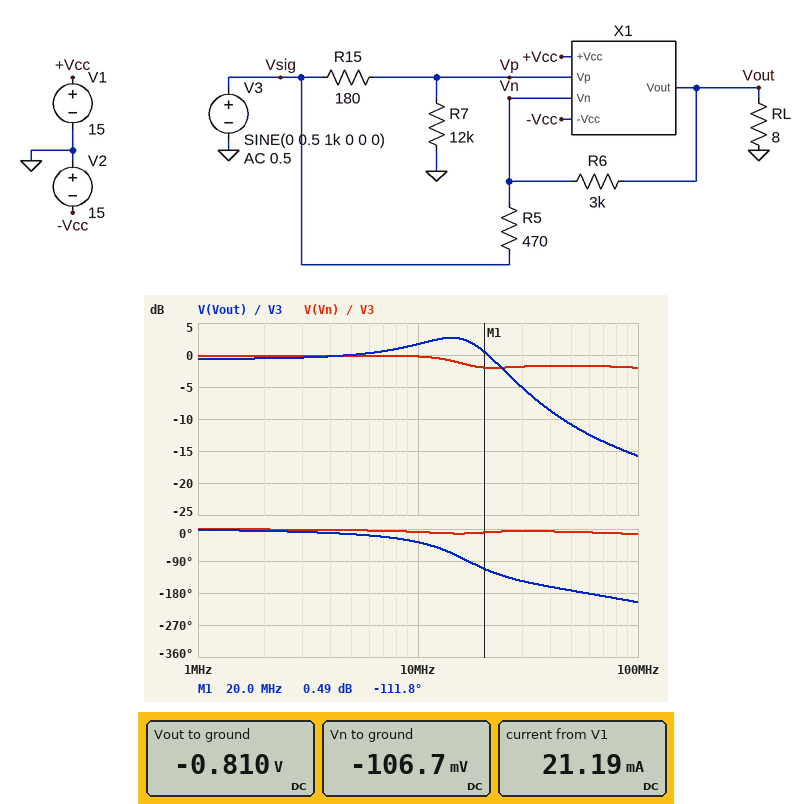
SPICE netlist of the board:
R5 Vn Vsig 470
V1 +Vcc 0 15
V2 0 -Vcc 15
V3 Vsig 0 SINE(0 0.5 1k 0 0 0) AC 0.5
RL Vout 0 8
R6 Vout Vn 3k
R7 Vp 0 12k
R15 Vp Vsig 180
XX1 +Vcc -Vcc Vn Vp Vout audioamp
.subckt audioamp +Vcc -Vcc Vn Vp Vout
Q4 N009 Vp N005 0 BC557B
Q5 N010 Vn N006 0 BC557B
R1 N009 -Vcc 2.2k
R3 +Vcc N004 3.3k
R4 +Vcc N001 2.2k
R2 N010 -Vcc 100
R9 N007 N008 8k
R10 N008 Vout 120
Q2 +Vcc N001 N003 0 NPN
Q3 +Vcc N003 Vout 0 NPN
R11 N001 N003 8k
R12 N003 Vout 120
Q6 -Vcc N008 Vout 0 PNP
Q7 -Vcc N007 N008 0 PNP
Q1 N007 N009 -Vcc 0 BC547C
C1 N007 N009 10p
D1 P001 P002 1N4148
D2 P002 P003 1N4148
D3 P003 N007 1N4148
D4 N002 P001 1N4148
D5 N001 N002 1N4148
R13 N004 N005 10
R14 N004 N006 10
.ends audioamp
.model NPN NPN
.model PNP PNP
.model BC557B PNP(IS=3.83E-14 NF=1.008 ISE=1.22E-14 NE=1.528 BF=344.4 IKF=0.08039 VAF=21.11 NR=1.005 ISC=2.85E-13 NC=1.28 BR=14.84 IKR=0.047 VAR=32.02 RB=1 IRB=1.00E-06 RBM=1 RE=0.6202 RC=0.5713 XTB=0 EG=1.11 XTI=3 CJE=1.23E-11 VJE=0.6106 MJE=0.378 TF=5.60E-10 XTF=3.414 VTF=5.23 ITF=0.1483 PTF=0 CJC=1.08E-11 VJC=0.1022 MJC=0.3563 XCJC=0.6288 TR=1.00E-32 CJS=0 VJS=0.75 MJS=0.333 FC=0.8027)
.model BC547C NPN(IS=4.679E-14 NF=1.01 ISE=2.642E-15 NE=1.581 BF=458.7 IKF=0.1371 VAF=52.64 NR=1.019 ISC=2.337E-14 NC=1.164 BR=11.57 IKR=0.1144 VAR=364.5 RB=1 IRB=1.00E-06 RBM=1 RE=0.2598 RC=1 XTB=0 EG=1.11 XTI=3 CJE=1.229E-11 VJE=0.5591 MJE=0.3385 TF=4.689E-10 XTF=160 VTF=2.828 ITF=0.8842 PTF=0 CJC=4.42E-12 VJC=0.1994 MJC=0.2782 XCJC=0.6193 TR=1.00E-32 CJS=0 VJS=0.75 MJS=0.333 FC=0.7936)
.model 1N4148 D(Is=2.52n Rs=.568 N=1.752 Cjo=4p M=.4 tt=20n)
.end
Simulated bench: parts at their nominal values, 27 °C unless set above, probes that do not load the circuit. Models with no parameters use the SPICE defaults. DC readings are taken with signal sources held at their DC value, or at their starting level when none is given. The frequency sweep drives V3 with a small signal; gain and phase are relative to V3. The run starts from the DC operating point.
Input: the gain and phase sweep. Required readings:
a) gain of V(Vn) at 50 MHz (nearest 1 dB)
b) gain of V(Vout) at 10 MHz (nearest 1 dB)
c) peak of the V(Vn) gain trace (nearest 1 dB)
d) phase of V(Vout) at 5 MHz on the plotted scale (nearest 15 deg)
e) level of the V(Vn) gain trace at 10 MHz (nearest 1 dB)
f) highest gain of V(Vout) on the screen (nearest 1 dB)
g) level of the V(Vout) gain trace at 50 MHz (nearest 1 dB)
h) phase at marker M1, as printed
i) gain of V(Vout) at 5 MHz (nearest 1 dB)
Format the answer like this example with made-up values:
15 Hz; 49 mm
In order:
-2 dB; 2 dB; 0 dB; -15 deg; 0 dB; 3 dB; -11 dB; -111.8 deg; 0 dB
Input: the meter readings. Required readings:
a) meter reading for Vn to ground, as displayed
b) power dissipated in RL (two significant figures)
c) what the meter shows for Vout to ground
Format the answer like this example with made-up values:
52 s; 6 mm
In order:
-106.7 mV; 82 mW; -0.810 V
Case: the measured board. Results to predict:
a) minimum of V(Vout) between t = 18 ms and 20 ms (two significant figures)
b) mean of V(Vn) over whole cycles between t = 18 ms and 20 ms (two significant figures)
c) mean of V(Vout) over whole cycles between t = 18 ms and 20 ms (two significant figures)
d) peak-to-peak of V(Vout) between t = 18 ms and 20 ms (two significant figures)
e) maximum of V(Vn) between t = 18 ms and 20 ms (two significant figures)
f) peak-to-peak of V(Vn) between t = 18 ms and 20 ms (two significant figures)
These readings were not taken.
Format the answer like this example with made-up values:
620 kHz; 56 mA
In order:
-1.3 V; -110 mV; -810 mV; 930 mV; 390 mV; 990 mV
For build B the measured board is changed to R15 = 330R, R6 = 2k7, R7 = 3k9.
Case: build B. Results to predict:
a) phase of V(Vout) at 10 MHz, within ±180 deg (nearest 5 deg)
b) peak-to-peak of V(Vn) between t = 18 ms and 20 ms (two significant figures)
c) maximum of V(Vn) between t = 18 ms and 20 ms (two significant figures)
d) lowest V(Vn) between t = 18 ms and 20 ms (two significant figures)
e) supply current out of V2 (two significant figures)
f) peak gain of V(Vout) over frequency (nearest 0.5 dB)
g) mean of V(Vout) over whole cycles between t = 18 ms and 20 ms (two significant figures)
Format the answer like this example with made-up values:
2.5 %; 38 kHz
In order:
-45 deg; 930 mV; 360 mV; -570 mV; 110 mA; -0.5 dB; -740 mV
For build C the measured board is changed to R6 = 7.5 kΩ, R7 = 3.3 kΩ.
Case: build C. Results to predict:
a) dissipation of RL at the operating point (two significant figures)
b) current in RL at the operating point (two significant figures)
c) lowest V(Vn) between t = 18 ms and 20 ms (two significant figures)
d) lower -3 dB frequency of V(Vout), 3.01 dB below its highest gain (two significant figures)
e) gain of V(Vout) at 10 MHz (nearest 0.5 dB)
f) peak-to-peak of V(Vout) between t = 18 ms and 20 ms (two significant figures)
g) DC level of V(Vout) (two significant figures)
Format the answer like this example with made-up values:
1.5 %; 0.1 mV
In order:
430 mW; 230 mA; -580 mV; 4.5 MHz; -7.5 dB; 210 mV; -1.9 V
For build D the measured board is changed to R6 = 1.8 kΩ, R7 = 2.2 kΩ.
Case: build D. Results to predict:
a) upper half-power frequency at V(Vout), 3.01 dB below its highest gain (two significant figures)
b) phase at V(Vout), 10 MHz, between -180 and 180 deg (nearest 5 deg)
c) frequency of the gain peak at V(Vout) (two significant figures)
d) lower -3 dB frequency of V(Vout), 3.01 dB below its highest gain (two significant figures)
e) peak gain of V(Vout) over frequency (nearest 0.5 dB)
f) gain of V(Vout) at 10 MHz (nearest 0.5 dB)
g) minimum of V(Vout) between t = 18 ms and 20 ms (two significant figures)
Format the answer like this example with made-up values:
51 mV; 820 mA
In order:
26 MHz; -20 deg; 19 MHz; 12 MHz; 2.0 dB; -1.5 dB; -860 mV
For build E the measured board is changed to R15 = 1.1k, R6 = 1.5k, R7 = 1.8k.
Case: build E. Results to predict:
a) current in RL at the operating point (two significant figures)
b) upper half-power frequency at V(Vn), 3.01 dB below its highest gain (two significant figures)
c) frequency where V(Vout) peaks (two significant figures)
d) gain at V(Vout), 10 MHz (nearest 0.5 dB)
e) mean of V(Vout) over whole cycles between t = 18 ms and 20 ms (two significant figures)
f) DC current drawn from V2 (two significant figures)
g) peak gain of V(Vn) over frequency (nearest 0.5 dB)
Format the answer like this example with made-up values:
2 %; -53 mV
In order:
57 mA; 140 MHz; 13 MHz; -0.5 dB; -460 mV; 80 mA; -2.0 dB
